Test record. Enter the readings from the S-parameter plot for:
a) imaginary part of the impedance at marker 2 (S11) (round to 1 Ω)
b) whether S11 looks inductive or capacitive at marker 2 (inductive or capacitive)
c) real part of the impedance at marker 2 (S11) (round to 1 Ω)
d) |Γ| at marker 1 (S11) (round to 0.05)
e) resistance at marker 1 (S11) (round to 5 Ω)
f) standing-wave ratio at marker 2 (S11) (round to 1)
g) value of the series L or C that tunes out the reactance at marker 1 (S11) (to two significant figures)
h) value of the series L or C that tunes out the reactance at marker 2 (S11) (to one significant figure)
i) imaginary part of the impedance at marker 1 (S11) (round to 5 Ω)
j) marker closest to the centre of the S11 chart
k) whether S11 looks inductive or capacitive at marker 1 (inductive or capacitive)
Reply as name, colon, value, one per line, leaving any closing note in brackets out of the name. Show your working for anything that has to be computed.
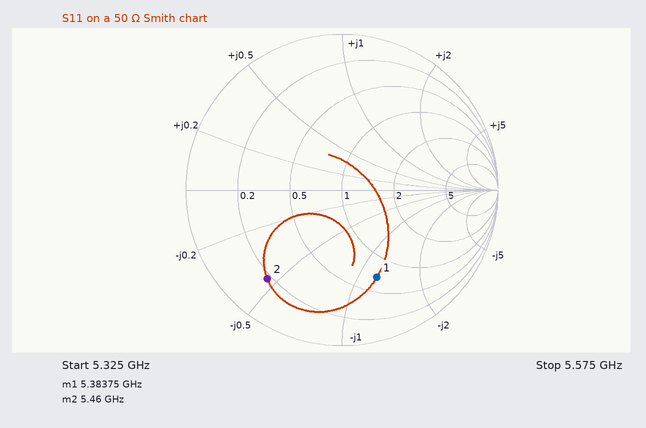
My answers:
imaginary part of the impedance at marker 2 (S11): -23 Ω
whether S11 looks inductive or capacitive at marker 2: capacitive
real part of the impedance at marker 2 (S11): 9 Ω
|Γ| at marker 1 (S11): 0.60
resistance at marker 1 (S11): 35 Ω
standing-wave ratio at marker 2 (S11): 7
value of the series L or C that tunes out the reactance at marker 1 (S11): L = 60 Ω/(2π × 5.38375 GHz) ≈ 1.8 nH
value of the series L or C that tunes out the reactance at marker 2 (S11): L = 23 Ω/(2π × 5.46 GHz) ≈ 670 pH, so 700 pH to one significant figure
imaginary part of the impedance at marker 1 (S11): -60 Ω
marker closest to the centre of the S11 chart: marker 1
whether S11 looks inductive or capacitive at marker 1: capacitive
